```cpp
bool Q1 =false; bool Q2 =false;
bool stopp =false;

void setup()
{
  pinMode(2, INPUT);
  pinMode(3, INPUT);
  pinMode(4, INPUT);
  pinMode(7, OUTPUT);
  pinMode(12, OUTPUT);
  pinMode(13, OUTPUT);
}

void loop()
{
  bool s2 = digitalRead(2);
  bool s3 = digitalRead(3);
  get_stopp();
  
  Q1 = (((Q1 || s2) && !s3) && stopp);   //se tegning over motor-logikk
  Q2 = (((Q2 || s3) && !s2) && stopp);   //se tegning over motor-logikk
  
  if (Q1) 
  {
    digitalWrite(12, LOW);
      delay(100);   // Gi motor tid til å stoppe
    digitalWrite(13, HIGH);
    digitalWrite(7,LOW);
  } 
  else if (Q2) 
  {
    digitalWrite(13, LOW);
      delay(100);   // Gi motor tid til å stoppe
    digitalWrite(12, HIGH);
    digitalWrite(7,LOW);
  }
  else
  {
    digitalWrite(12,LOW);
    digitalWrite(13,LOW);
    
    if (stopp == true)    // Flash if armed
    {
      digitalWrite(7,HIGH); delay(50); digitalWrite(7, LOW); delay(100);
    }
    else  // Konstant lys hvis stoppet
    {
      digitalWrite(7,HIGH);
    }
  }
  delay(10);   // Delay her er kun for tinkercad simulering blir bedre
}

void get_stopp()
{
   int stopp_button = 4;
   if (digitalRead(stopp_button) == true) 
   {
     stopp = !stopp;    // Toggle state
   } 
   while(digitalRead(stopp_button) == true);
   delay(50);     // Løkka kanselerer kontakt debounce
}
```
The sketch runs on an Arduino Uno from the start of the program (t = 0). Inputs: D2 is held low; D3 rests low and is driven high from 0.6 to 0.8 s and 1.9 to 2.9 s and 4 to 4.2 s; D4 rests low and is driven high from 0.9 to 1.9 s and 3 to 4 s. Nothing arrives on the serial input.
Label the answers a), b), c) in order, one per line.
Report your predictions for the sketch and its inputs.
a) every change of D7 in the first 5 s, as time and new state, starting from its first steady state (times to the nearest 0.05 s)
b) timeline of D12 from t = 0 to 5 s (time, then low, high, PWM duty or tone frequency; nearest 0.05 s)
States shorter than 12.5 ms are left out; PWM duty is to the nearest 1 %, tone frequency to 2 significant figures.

a) 0 s low; 0.05 s high; 2 s low; 4.05 s high
b) 0 s low; 2.25 s high; 4.05 s low
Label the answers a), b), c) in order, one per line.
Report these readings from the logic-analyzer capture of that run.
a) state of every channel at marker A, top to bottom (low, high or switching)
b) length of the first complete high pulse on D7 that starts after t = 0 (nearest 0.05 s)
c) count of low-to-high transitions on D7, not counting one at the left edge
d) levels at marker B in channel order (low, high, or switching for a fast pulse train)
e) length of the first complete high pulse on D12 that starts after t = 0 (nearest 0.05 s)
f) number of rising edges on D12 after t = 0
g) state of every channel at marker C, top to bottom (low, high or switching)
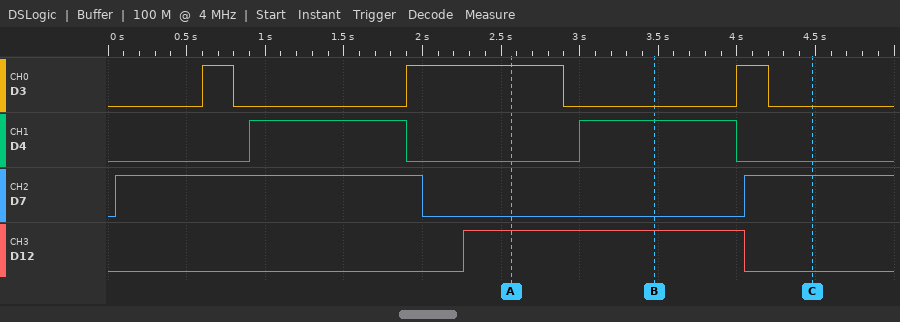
a) D3 high, D4 low, D7 low, D12 high
b) 1.95 s
c) 2
d) D3 low, D4 high, D7 low, D12 high
e) 1.80 s
f) 1
g) D3 low, D4 low, D7 high, D12 low
